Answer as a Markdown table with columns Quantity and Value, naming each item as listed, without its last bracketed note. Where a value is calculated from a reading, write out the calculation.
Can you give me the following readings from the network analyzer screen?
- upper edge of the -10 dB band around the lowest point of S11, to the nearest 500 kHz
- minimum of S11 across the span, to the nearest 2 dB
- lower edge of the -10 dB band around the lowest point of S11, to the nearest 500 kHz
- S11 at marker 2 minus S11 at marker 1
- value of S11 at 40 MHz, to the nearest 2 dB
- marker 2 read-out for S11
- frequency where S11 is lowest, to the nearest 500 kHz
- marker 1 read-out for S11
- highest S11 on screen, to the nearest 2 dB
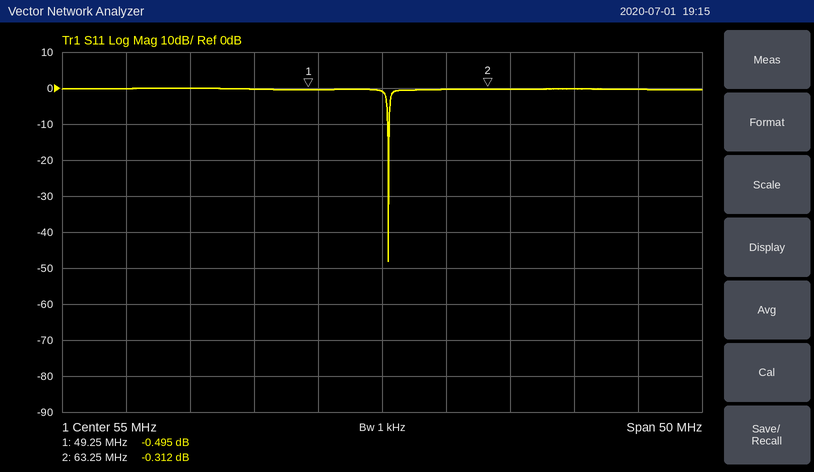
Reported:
| Quantity | Value |
|---|---|
| upper edge of the -10 dB band around the lowest point of S11, to the nearest 500 kHz | 55.5 MHz |
| minimum of S11 across the span, to the nearest 2 dB | -48 dB |
| lower edge of the -10 dB band around the lowest point of S11, to the nearest 500 kHz | 55.5 MHz |
| S11 at marker 2 minus S11 at marker 1 | -0.312 − (-0.495) = 0.183 dB |
| value of S11 at 40 MHz, to the nearest 2 dB | 0 dB |
| marker 2 read-out for S11 | -0.312 dB |
| frequency where S11 is lowest, to the nearest 500 kHz | 55.5 MHz |
| marker 1 read-out for S11 | -0.495 dB |
| highest S11 on screen, to the nearest 2 dB | 0 dB |
